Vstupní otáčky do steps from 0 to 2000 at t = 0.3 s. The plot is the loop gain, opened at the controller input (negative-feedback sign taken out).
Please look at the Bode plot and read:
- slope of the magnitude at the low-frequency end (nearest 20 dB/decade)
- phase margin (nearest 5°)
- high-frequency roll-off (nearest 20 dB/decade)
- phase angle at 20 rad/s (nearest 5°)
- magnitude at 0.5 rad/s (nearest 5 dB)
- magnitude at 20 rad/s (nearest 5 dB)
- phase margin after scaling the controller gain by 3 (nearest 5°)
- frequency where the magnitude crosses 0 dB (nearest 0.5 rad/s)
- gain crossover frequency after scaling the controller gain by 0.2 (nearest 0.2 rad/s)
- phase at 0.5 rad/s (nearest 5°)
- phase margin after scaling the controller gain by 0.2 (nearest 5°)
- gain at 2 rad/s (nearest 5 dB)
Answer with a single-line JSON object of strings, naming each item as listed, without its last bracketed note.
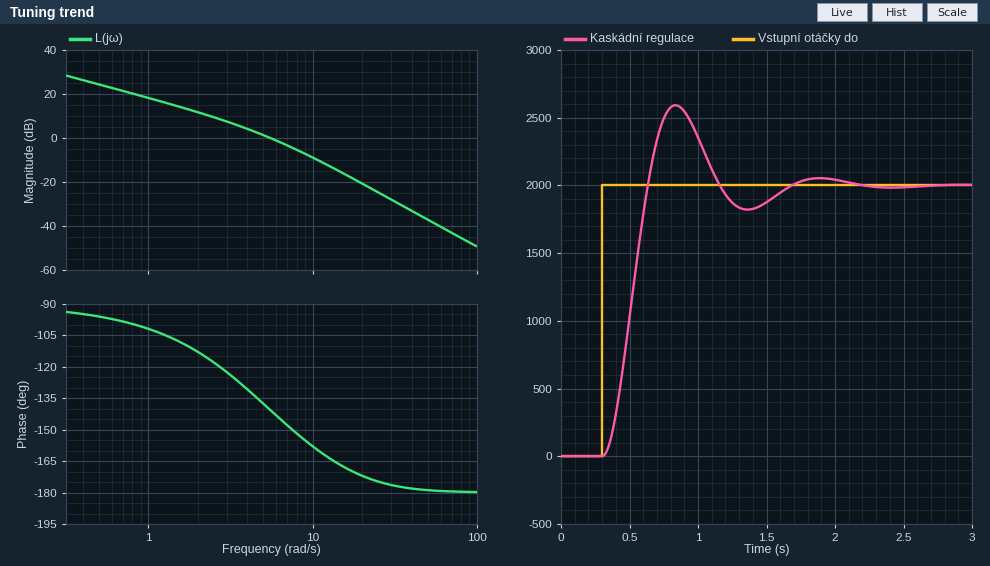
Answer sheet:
{"slope of the magnitude at the low-frequency end": "-20 dB/decade", "phase margin": "40°", "high-frequency roll-off": "-40 dB/decade", "phase angle at 20 rad/s": "-170°", "magnitude at 0.5 rad/s": "25 dB", "magnitude at 20 rad/s": "-20 dB", "phase margin after scaling the controller gain by 3": "20°", "frequency where the magnitude crosses 0 dB": "5.5 rad/s", "gain crossover frequency after scaling the controller gain by 0.2": "1.6 rad/s", "phase at 0.5 rad/s": "-95°", "phase margin after scaling the controller gain by 0.2": "70°", "gain at 2 rad/s": "10 dB"}
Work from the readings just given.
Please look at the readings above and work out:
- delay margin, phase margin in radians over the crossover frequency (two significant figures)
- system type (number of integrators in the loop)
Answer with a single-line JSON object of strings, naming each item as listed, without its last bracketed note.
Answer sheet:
{"delay margin, phase margin in radians over the crossover frequency": "0.13 s", "system type": "1"}
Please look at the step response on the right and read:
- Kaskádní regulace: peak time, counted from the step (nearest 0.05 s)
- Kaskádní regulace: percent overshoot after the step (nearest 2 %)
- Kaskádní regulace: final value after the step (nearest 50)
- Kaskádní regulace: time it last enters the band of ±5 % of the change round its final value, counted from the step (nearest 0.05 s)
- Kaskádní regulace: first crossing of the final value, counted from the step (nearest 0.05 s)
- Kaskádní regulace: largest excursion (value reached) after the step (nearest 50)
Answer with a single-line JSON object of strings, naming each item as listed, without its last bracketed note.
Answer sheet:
{"Kaskádní regulace: peak time, counted from the step": "0.55 s", "Kaskádní regulace: percent overshoot after the step": "30 %", "Kaskádní regulace: final value after the step": "2000", "Kaskádní regulace: time it last enters the band of ±5 % of the change round its final value, counted from the step": "1.25 s", "Kaskádní regulace: first crossing of the final value, counted from the step": "0.35 s", "Kaskádní regulace: largest excursion (value reached) after the step": "2600"}
